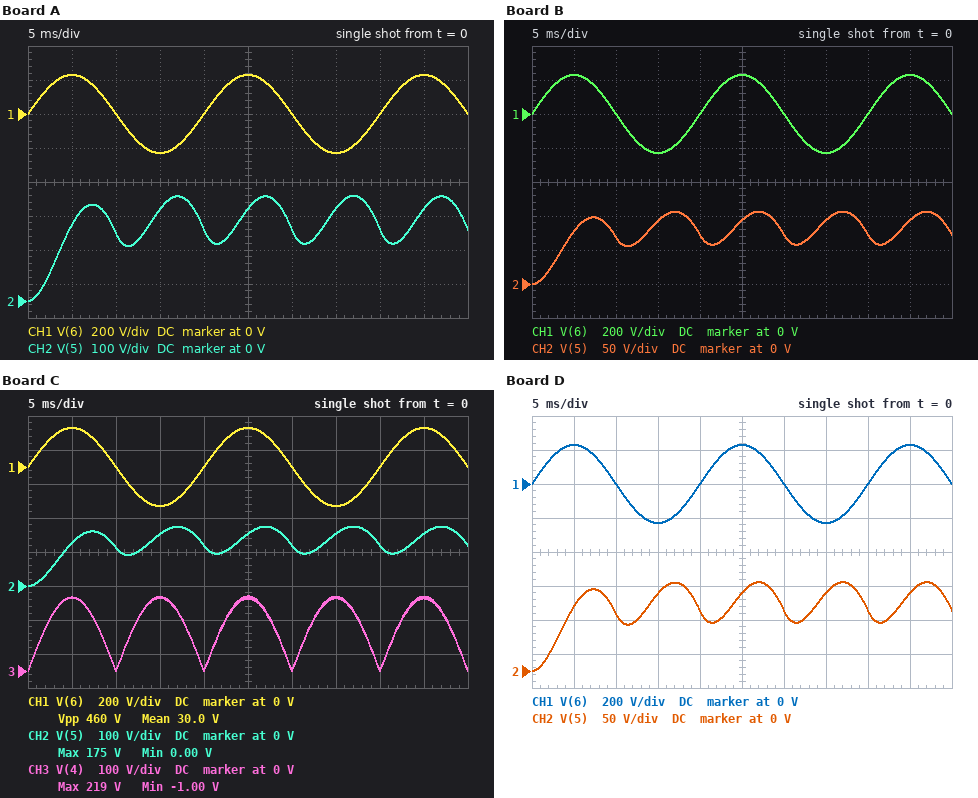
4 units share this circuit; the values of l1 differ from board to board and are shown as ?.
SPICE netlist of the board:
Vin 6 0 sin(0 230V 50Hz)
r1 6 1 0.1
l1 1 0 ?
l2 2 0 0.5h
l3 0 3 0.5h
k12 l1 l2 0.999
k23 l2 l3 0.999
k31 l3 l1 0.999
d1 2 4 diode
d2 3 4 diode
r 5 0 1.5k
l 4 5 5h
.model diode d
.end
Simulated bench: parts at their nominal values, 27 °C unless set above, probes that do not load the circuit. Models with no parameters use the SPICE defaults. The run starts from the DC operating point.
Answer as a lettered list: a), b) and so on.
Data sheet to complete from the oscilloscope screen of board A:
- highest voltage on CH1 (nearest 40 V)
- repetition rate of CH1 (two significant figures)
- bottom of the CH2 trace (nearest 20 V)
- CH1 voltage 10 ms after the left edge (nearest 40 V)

a) 240 V
b) 50 Hz
c) 0 V
d) 0 V
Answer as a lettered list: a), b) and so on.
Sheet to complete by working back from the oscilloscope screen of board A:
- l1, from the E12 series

a) 180 mH
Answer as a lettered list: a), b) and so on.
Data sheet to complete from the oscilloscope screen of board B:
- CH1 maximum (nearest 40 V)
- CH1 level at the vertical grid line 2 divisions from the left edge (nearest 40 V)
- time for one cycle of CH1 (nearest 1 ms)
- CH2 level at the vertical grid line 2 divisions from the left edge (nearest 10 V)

a) 240 V
b) 0 V
c) 20 ms
d) 70 V
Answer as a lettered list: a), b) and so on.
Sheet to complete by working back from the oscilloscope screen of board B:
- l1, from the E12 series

a) 1.5 H
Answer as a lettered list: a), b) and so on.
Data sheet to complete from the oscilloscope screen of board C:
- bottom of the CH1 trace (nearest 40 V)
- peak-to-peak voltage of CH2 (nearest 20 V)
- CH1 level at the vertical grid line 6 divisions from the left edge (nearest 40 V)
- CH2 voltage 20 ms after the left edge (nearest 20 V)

a) -240 V
b) 180 V
c) 0 V
d) 120 V
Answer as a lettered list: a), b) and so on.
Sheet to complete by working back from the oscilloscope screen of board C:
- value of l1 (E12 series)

a) 560 mH
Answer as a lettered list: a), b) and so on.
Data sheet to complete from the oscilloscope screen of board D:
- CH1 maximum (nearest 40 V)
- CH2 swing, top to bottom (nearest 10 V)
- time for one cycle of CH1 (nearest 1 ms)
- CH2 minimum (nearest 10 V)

a) 240 V
b) 130 V
c) 20 ms
d) 0 V
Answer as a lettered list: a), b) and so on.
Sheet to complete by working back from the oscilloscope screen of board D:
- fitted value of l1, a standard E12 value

a) 1 H
